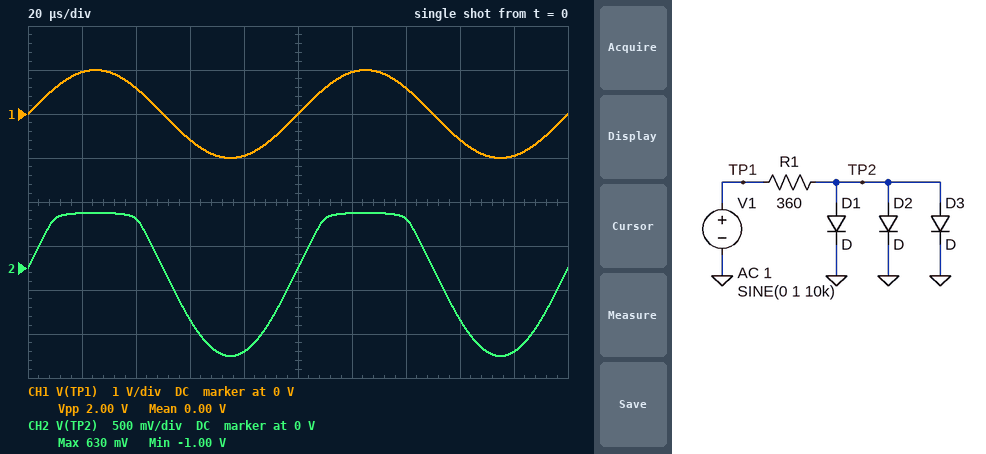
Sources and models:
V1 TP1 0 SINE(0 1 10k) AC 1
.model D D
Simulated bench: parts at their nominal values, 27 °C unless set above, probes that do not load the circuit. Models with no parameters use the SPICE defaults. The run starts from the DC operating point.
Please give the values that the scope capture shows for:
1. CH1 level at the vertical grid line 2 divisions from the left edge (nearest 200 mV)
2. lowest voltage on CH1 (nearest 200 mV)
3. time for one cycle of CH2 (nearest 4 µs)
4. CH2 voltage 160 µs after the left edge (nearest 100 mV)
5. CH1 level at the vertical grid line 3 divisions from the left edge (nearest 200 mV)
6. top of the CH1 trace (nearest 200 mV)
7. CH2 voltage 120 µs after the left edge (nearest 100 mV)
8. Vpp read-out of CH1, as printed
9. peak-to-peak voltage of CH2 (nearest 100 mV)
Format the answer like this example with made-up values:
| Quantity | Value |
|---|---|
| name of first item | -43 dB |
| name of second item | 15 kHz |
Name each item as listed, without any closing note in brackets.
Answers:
| Quantity | Value |
|---|---|
| CH1 level at the vertical grid line 2 divisions from the left edge | 600 mV |
| lowest voltage on CH1 | -1.0 V |
| time for one cycle of CH2 | 100 µs |
| CH2 voltage 160 µs after the left edge | -600 mV |
| CH1 level at the vertical grid line 3 divisions from the left edge | -600 mV |
| top of the CH1 trace | 1.0 V |
| CH2 voltage 120 µs after the left edge | 600 mV |
| Vpp read-out of CH1, as printed | 2.00 V |
| peak-to-peak voltage of CH2 | 1.6 V |
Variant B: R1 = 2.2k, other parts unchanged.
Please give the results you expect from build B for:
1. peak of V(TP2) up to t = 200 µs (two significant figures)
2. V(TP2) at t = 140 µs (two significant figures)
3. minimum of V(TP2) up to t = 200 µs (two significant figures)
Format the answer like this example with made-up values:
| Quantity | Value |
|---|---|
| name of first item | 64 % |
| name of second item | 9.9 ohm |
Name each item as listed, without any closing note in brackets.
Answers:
| Quantity | Value |
|---|---|
| peak of V(TP2) up to t = 200 µs | 580 mV |
| V(TP2) at t = 140 µs | 530 mV |
| minimum of V(TP2) up to t = 200 µs | -1.0 V |
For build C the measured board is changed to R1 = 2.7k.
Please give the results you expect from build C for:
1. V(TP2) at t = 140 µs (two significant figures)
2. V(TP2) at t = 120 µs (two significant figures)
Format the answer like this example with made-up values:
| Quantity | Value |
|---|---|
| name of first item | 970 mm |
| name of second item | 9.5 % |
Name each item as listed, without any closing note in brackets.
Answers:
| Quantity | Value |
|---|---|
| V(TP2) at t = 140 µs | 530 mV |
| V(TP2) at t = 120 µs | 580 mV |
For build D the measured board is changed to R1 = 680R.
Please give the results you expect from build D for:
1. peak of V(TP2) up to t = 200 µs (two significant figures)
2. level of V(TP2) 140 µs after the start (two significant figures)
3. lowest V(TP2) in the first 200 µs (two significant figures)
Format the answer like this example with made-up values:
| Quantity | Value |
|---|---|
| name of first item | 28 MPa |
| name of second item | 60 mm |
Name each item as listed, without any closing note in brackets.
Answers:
| Quantity | Value |
|---|---|
| peak of V(TP2) up to t = 200 µs | 610 mV |
| level of V(TP2) 140 µs after the start | 550 mV |
| lowest V(TP2) in the first 200 µs | -1.0 V |
